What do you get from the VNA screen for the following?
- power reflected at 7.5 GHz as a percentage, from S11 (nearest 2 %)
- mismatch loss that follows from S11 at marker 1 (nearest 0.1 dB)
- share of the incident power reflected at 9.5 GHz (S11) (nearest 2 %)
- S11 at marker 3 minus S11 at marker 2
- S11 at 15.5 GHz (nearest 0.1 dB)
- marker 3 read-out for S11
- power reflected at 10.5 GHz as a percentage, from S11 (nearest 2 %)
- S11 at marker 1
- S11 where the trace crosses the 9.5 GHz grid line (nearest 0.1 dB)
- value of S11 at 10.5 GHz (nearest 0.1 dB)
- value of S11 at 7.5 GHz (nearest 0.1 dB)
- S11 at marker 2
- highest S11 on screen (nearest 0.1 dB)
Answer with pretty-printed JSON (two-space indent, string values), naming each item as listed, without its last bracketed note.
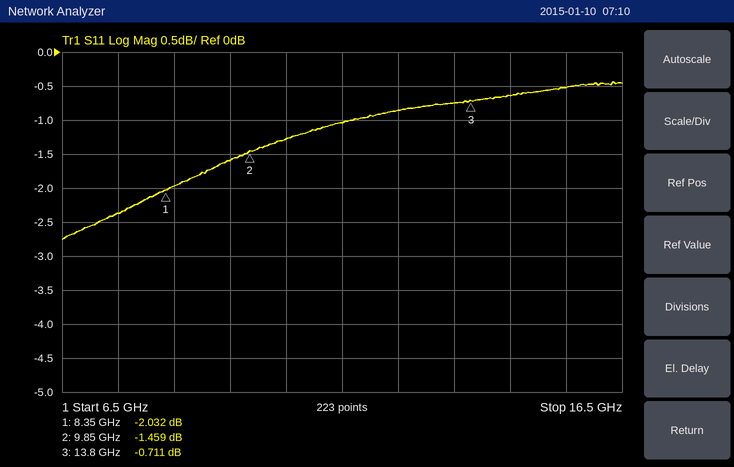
{
  "power reflected at 7.5 GHz as a percentage, from S11": "58 %",
  "mismatch loss that follows from S11 at marker 1": "4.3 dB",
  "share of the incident power reflected at 9.5 GHz (S11)": "70 %",
  "S11 at marker 3 minus S11 at marker 2": "0.748 dB",
  "S11 at 15.5 GHz": "-0.5 dB",
  "marker 3 read-out for S11": "-0.711 dB",
  "power reflected at 10.5 GHz as a percentage, from S11": "74 %",
  "S11 at marker 1": "-2.032 dB",
  "S11 where the trace crosses the 9.5 GHz grid line": "-1.6 dB",
  "value of S11 at 10.5 GHz": "-1.3 dB",
  "value of S11 at 7.5 GHz": "-2.4 dB",
  "S11 at marker 2": "-1.459 dB",
  "highest S11 on screen": "-0.4 dB"
}
